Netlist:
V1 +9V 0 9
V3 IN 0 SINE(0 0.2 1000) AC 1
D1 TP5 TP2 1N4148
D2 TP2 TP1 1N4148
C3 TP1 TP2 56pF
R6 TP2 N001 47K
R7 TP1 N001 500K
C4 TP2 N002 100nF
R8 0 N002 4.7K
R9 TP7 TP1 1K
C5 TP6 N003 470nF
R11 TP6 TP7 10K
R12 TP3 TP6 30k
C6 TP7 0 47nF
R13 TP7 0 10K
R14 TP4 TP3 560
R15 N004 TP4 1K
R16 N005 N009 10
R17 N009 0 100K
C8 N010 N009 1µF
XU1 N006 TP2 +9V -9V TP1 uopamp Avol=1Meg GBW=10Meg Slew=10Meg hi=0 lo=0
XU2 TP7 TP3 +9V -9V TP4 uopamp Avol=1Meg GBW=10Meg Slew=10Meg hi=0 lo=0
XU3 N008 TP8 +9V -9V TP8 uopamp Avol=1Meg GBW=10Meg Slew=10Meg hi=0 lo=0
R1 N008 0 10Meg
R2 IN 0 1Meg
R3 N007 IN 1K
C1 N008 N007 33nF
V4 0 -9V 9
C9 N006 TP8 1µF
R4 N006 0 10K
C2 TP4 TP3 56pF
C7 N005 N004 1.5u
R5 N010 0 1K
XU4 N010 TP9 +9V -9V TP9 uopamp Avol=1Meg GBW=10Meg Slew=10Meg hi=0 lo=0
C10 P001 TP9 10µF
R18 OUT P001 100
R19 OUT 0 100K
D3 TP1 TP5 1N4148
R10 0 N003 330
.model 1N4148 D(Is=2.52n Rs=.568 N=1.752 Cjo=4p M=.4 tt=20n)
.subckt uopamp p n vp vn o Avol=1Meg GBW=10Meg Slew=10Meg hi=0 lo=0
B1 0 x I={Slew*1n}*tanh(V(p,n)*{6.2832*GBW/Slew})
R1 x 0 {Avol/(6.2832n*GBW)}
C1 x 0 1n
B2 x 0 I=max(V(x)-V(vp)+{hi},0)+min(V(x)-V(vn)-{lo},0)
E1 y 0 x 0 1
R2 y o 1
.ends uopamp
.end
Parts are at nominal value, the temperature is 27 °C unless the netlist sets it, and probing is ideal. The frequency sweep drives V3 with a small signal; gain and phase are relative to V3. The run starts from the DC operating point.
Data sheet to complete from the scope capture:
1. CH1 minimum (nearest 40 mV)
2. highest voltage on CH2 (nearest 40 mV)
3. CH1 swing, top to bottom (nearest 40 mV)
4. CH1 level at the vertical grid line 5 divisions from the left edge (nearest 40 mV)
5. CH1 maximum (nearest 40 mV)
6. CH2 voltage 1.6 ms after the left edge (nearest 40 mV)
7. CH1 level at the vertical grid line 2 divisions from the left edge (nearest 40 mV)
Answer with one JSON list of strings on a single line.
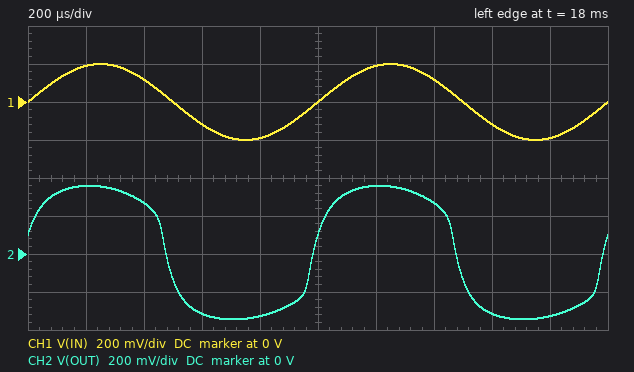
["-200 mV", "360 mV", "400 mV", "0 V", "200 mV", "-320 mV", "120 mV"]
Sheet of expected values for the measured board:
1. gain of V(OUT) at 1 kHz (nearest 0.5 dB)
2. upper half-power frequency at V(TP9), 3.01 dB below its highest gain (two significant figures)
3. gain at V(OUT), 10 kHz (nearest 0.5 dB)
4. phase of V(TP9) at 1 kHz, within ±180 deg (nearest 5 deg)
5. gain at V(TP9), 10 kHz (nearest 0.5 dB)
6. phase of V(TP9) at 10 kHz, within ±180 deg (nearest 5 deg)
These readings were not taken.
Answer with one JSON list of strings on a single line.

["32.5 dB", "3.3 kHz", "17.5 dB", "0 deg", "17.5 dB", "-130 deg"]
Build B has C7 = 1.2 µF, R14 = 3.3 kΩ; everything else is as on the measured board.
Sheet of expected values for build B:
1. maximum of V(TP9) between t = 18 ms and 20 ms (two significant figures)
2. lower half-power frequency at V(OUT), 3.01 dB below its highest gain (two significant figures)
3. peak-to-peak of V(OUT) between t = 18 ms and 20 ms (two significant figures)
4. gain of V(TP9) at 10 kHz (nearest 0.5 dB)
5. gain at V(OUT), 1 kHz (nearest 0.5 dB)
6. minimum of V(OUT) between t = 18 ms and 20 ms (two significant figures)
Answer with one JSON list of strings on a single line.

["390 mV", "330 Hz", "760 mV", "18.0 dB", "33.0 dB", "-370 mV"]
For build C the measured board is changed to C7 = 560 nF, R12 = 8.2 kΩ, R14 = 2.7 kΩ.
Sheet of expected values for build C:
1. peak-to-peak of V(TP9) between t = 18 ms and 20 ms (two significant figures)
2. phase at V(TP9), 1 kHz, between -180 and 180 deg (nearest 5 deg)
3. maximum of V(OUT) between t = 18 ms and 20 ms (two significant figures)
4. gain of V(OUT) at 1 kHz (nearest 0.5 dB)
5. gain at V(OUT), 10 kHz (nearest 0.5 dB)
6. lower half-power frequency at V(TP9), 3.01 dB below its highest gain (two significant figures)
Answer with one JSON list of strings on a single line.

["910 mV", "5 deg", "460 mV", "34.5 dB", "19.5 dB", "370 Hz"]
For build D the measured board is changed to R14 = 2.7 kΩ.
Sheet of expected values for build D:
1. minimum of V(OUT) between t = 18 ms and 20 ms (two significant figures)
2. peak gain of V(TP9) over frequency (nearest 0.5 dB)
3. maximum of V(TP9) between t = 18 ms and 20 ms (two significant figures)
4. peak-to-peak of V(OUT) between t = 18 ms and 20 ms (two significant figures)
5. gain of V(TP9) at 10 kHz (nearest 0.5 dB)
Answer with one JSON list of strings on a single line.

["-370 mV", "33.0 dB", "380 mV", "750 mV", "18.0 dB"]
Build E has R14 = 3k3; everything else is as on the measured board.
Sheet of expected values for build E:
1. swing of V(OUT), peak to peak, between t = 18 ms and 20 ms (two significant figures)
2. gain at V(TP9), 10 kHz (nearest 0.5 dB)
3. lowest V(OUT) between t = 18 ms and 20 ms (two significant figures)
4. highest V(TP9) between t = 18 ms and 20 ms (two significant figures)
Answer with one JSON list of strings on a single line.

["760 mV", "18.0 dB", "-370 mV", "390 mV"]
